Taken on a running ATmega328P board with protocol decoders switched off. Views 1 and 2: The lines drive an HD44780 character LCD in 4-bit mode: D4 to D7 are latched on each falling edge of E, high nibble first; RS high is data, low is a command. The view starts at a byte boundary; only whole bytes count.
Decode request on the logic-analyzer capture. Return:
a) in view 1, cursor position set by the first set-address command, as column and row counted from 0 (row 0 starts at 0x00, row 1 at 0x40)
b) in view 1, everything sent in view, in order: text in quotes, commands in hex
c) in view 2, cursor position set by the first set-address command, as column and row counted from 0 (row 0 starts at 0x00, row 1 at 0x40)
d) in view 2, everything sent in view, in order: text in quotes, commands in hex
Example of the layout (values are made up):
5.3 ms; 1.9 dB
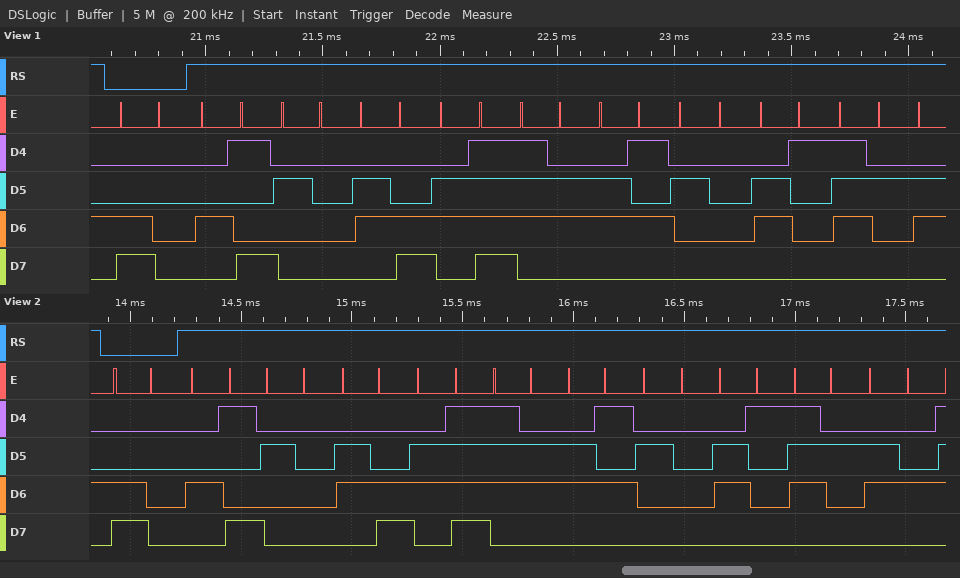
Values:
column 0, row 1; 0xC0 "I love ar"; column 0, row 1; 0xC0 "I love ard"
